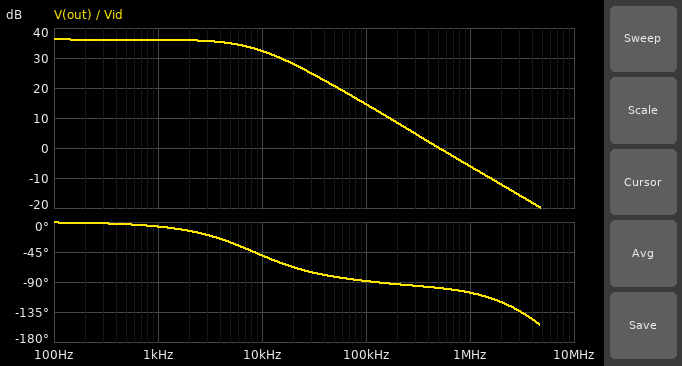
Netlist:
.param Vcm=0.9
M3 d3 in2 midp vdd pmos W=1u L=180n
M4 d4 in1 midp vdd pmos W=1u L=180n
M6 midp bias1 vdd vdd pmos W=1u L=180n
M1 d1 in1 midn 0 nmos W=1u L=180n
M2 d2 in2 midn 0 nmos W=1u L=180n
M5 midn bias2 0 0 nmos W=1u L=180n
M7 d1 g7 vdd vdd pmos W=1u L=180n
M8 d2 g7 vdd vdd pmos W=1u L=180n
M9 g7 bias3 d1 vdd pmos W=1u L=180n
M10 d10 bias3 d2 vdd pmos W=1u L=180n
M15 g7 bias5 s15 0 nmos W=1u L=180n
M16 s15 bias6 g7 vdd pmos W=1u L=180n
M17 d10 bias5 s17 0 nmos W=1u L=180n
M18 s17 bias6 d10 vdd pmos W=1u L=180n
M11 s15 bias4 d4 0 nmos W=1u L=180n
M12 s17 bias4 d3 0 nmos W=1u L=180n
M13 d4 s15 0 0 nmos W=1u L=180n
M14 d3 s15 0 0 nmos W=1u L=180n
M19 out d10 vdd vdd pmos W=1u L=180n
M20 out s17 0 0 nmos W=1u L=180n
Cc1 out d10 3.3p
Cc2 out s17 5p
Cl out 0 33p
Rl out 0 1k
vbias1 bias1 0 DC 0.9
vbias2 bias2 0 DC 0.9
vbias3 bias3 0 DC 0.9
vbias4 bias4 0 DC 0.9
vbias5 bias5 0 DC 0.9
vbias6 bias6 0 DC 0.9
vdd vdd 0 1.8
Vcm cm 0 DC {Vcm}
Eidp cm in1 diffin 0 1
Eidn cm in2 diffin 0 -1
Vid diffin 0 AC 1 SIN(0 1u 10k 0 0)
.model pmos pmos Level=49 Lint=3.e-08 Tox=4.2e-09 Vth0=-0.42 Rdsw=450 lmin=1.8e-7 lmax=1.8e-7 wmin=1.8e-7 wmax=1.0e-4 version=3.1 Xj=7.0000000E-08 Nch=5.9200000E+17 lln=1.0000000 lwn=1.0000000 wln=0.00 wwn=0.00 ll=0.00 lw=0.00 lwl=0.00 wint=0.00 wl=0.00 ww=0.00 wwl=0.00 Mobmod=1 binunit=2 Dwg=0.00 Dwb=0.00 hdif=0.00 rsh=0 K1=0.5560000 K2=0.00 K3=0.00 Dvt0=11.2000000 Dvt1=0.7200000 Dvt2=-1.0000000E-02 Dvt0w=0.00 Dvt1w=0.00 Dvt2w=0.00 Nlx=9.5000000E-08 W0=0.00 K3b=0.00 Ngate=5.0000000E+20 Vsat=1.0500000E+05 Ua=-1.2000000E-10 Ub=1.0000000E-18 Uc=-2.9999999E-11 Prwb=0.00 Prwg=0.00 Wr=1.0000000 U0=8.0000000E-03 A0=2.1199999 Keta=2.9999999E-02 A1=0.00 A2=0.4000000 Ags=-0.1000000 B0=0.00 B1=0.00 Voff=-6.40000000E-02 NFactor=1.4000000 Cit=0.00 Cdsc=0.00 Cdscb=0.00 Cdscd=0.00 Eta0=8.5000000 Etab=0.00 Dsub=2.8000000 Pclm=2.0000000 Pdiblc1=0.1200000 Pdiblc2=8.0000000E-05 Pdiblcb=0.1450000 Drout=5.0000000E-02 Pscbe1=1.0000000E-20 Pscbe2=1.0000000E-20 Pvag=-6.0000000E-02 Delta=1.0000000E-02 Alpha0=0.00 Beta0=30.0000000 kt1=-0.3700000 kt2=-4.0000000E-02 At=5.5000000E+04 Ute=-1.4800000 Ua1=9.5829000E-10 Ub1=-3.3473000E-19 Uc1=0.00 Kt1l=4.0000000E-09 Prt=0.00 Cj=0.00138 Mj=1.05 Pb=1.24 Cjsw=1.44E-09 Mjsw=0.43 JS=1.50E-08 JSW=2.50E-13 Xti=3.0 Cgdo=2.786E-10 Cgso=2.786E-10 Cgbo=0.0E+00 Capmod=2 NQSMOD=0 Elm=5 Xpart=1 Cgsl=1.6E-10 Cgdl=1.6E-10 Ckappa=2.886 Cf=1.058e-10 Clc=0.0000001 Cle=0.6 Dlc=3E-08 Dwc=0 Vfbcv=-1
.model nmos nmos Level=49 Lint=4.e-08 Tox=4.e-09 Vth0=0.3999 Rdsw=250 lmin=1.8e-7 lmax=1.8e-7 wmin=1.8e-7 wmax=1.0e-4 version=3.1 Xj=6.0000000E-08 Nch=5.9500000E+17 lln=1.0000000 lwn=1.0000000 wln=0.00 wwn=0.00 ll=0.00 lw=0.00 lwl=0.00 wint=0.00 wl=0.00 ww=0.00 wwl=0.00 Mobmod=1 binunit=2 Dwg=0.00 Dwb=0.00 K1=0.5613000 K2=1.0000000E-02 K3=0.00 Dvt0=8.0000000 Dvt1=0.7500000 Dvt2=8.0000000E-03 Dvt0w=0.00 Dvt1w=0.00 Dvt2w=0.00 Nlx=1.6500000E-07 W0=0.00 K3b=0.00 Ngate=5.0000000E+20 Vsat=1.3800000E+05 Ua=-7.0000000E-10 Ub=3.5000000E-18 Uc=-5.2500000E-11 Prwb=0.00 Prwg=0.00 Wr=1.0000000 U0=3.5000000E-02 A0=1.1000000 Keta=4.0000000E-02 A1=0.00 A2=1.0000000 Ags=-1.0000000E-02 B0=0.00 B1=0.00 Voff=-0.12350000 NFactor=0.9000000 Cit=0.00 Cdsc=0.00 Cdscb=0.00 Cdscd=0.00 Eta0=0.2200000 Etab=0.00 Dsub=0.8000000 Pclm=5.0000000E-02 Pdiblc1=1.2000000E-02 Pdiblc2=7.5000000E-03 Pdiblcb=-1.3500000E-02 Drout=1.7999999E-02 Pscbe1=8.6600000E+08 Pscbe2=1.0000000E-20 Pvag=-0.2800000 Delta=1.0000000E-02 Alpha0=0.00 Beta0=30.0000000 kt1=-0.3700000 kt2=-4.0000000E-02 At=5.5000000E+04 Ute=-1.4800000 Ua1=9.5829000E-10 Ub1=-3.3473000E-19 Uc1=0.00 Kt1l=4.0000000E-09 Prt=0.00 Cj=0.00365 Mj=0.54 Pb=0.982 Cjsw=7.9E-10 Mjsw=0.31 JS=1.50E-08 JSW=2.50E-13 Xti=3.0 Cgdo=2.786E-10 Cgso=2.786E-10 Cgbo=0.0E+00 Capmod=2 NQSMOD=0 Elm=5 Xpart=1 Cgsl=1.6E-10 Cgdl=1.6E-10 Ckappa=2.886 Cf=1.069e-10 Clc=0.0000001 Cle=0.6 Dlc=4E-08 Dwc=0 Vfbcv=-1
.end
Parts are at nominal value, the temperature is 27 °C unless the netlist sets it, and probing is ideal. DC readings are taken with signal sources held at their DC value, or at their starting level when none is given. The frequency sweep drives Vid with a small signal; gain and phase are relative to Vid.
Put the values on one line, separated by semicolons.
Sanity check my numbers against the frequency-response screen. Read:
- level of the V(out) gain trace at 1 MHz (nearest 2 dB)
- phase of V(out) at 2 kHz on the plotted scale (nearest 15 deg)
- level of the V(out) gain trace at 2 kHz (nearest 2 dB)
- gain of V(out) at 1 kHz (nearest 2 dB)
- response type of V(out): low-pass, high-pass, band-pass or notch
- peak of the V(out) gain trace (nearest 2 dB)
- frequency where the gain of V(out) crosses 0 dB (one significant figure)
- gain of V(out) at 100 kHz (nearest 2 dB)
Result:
-6 dB; -15 deg; 36 dB; 36 dB; low-pass; 36 dB; 500 kHz; 14 dB
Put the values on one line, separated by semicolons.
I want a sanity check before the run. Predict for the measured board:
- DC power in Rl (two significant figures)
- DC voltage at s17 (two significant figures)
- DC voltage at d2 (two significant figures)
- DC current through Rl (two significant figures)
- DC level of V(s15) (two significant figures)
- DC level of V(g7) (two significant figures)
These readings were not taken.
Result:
7.7 µW; 550 mV; 1.2 V; 88 µA; 550 mV; 930 mV
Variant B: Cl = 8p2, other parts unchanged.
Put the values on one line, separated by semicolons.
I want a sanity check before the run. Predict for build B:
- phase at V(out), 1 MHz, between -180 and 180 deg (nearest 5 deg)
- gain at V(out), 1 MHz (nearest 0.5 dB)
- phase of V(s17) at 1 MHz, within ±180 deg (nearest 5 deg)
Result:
-100 deg; -6.0 dB; 105 deg
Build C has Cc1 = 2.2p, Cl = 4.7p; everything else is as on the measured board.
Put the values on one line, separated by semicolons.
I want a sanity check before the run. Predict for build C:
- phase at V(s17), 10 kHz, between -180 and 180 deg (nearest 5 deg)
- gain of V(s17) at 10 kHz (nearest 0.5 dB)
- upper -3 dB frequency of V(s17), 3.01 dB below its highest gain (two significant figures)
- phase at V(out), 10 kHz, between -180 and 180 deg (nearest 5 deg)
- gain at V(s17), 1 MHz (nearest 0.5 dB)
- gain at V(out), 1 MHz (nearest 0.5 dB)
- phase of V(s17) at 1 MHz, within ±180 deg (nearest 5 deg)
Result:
145 deg; 23.5 dB; 12 kHz; -40 deg; -2.0 dB; -3.5 dB; 105 deg
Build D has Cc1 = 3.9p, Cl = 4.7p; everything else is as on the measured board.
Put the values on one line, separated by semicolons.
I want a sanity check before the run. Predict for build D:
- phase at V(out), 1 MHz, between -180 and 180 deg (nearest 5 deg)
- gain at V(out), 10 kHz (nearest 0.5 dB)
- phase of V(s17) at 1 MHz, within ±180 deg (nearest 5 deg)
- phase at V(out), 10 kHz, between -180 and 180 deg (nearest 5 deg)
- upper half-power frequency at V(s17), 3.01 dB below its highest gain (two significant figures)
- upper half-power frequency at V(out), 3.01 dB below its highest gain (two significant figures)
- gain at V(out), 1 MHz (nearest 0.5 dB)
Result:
-100 deg; 31.5 dB; 105 deg; -55 deg; 7.8 kHz; 7.4 kHz; -7.0 dB
